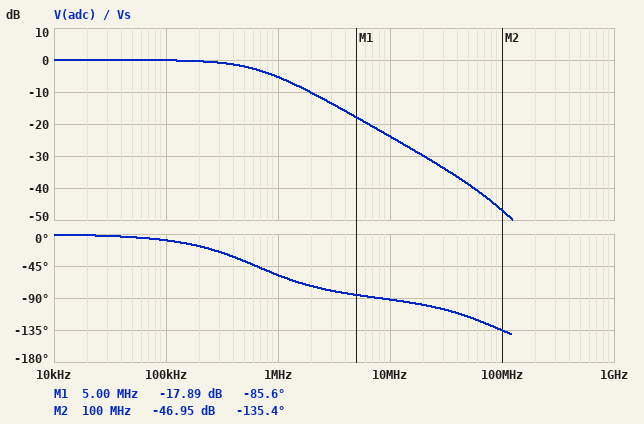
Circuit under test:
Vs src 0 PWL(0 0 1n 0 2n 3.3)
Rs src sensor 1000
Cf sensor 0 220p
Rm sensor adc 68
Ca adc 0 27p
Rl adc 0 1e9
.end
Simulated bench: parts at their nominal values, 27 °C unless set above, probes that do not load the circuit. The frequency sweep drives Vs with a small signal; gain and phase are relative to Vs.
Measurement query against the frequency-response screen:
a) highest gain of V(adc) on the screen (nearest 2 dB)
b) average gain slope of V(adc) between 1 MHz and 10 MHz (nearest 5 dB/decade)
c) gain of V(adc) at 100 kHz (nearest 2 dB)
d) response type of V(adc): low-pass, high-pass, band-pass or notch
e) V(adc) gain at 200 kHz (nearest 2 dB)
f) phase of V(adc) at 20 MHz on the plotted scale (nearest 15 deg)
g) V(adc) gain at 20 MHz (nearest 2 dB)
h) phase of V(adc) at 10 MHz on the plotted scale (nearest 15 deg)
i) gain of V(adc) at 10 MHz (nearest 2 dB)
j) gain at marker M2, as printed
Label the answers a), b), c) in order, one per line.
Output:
a) 0 dB
b) -20 dB/decade
c) 0 dB
d) low-pass
e) 0 dB
f) -105 deg
g) -30 dB
h) -90 deg
i) -24 dB
j) -46.95 dB
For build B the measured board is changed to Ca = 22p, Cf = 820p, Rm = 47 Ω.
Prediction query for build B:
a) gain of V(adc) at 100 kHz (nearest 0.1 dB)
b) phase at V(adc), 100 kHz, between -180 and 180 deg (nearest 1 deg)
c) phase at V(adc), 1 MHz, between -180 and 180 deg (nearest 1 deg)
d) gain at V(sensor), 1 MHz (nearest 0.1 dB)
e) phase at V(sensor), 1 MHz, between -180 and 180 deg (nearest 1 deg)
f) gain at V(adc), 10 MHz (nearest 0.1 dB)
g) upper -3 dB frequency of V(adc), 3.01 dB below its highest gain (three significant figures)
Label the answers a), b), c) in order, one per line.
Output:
a) -1.1 dB
b) -28 deg
c) -80 deg
d) -14.6 dB
e) -79 deg
f) -34.5 dB
g) 189 kHz
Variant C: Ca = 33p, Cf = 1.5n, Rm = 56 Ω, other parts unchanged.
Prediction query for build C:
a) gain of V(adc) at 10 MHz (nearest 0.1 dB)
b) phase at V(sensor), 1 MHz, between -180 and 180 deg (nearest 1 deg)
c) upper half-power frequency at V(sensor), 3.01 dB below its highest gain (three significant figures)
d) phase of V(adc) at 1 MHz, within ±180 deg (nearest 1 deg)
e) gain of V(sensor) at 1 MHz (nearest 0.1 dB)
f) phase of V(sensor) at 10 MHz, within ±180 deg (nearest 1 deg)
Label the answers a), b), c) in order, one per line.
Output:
a) -39.7 dB
b) -84 deg
c) 104 kHz
d) -85 deg
e) -19.7 dB
f) -89 deg
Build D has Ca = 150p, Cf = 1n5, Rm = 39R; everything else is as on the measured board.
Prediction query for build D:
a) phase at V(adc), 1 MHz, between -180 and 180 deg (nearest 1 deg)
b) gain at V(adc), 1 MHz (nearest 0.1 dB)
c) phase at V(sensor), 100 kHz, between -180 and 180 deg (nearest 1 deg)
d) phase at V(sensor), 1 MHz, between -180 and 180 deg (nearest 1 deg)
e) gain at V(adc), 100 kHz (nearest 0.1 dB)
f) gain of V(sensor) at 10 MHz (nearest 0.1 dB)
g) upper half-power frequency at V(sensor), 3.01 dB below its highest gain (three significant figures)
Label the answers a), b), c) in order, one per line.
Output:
a) -86 deg
b) -20.4 dB
c) -46 deg
d) -84 deg
e) -3.2 dB
f) -40.2 dB
g) 96.4 kHz
